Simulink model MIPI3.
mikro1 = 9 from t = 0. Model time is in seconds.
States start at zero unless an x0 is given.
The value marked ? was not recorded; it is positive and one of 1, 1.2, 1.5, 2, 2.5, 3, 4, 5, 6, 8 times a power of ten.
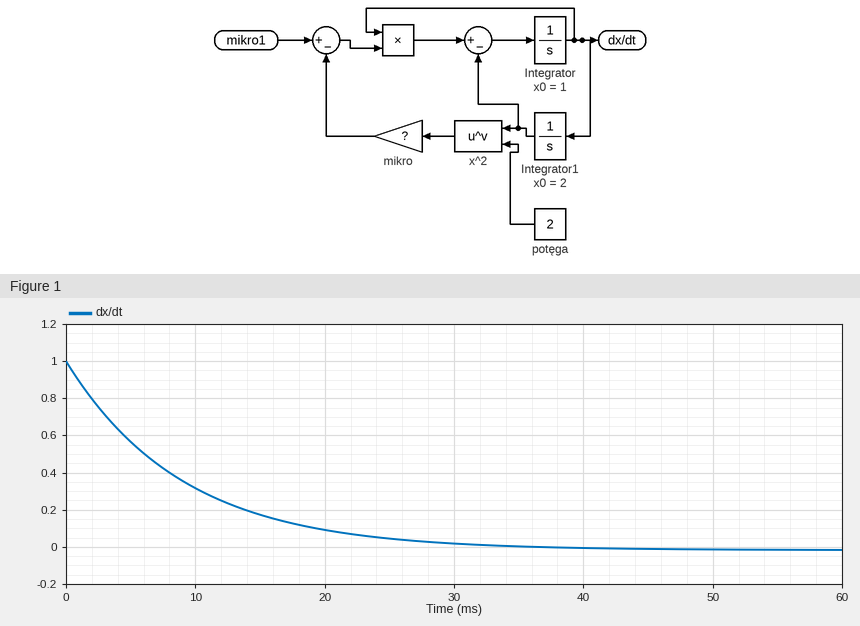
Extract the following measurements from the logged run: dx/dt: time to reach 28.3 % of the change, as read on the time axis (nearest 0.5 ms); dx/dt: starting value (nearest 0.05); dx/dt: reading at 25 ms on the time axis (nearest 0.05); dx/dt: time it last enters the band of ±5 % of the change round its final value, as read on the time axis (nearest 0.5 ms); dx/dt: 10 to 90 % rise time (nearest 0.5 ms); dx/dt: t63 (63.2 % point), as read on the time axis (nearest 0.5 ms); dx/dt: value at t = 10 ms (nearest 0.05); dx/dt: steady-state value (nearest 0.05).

3.0 ms
1.00
0.05
27.0 ms
19.5 ms
9.0 ms
0.30
0.00
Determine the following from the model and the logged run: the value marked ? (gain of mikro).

30
